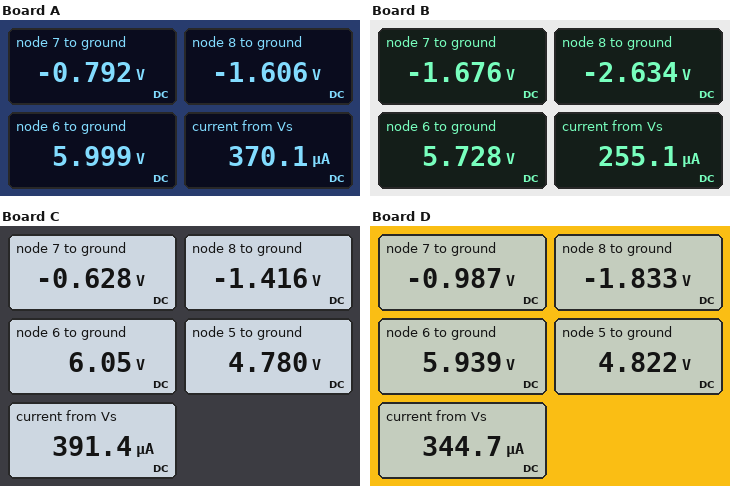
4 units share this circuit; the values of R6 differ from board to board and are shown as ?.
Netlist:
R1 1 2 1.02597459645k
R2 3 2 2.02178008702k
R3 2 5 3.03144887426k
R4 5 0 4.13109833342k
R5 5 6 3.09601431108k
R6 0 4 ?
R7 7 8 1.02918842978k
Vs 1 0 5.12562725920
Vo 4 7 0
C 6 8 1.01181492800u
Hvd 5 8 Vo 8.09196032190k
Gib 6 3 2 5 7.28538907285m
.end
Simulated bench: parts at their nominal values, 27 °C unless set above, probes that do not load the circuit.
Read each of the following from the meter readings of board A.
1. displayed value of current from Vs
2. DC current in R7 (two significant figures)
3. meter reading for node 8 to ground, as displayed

370.1 µA
790 µA
-1.606 V
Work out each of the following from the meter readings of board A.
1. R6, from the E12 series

1 kΩ
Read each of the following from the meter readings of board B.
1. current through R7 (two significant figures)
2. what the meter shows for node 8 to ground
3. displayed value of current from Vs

930 µA
-2.634 V
255.1 µA
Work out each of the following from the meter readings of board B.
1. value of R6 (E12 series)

1.8 kΩ
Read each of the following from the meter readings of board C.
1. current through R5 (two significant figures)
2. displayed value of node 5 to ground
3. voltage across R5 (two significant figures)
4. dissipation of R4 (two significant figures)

410 µA
4.780 V
1.3 V
5.5 mW
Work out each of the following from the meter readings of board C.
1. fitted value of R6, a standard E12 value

820 Ω
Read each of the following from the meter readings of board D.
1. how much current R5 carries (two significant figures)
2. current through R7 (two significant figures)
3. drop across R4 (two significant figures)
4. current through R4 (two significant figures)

360 µA
820 µA
4.8 V
1.2 mA
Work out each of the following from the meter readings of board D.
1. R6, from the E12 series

1.2 kΩ
